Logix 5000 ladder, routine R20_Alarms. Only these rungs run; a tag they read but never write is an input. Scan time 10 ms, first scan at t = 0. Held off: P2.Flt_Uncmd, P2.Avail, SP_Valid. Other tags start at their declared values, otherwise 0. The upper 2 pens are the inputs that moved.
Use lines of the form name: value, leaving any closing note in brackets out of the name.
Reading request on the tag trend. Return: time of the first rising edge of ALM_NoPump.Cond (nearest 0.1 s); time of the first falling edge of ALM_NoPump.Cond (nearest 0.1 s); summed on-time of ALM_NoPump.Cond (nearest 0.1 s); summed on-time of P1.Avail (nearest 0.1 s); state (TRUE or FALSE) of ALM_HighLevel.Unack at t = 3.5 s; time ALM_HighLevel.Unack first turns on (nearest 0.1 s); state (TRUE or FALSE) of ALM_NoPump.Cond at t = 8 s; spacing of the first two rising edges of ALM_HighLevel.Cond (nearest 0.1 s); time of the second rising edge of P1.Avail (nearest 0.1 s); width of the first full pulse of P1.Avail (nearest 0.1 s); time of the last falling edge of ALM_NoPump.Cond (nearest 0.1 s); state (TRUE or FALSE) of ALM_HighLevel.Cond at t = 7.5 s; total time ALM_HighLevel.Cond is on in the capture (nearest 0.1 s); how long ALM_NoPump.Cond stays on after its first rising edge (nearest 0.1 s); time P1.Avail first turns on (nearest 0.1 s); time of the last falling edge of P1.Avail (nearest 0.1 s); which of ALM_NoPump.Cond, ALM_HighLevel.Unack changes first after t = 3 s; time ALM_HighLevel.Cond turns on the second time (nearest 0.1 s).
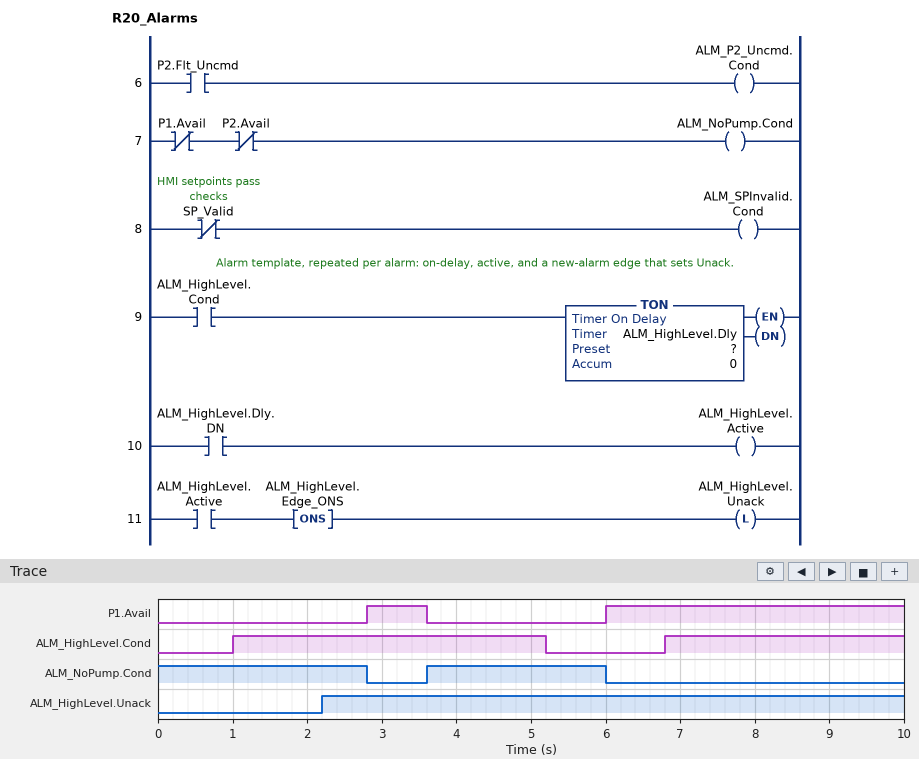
time of the first rising edge of ALM_NoPump.Cond: 3.6 s
time of the first falling edge of ALM_NoPump.Cond: 2.8 s
summed on-time of ALM_NoPump.Cond: 5.2 s
summed on-time of P1.Avail: 4.8 s
state (TRUE or FALSE) of ALM_HighLevel.Unack at t = 3.5 s: TRUE
time ALM_HighLevel.Unack first turns on: 2.2 s
state (TRUE or FALSE) of ALM_NoPump.Cond at t = 8 s: FALSE
spacing of the first two rising edges of ALM_HighLevel.Cond: 5.8 s
time of the second rising edge of P1.Avail: 6.0 s
width of the first full pulse of P1.Avail: 0.8 s
time of the last falling edge of ALM_NoPump.Cond: 6.0 s
state (TRUE or FALSE) of ALM_HighLevel.Cond at t = 7.5 s: TRUE
total time ALM_HighLevel.Cond is on in the capture: 7.4 s
how long ALM_NoPump.Cond stays on after its first rising edge: 2.4 s
time P1.Avail first turns on: 2.8 s
time of the last falling edge of P1.Avail: 3.6 s
which of ALM_NoPump.Cond, ALM_HighLevel.Unack changes first after t = 3 s: ALM_NoPump.Cond
time ALM_HighLevel.Cond turns on the second time: 6.8 s
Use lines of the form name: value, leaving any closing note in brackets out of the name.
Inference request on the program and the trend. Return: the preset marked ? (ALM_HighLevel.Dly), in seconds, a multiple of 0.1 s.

the preset marked ? (ALM_HighLevel.Dly), in seconds, a multiple of 0.1 s: 1.2 s
